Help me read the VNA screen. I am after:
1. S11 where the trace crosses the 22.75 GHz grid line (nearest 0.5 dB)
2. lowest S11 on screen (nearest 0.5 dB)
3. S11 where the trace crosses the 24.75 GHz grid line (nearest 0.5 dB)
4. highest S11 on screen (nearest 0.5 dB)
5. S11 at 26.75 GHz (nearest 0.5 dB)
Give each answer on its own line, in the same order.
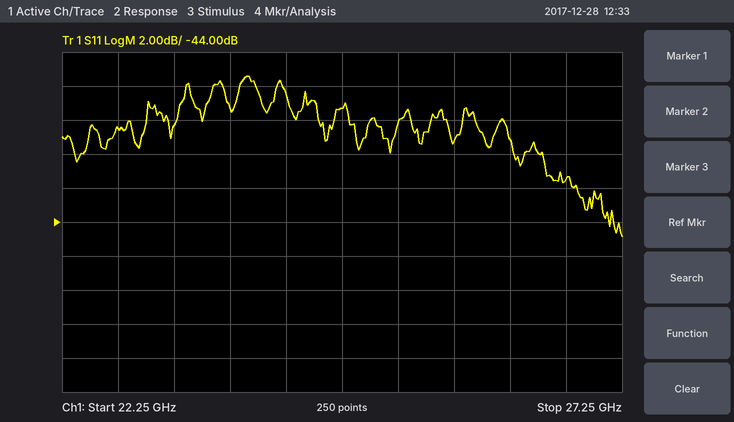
-38.5 dB
-45.0 dB
-37.5 dB
-35.5 dB
-41.5 dB
